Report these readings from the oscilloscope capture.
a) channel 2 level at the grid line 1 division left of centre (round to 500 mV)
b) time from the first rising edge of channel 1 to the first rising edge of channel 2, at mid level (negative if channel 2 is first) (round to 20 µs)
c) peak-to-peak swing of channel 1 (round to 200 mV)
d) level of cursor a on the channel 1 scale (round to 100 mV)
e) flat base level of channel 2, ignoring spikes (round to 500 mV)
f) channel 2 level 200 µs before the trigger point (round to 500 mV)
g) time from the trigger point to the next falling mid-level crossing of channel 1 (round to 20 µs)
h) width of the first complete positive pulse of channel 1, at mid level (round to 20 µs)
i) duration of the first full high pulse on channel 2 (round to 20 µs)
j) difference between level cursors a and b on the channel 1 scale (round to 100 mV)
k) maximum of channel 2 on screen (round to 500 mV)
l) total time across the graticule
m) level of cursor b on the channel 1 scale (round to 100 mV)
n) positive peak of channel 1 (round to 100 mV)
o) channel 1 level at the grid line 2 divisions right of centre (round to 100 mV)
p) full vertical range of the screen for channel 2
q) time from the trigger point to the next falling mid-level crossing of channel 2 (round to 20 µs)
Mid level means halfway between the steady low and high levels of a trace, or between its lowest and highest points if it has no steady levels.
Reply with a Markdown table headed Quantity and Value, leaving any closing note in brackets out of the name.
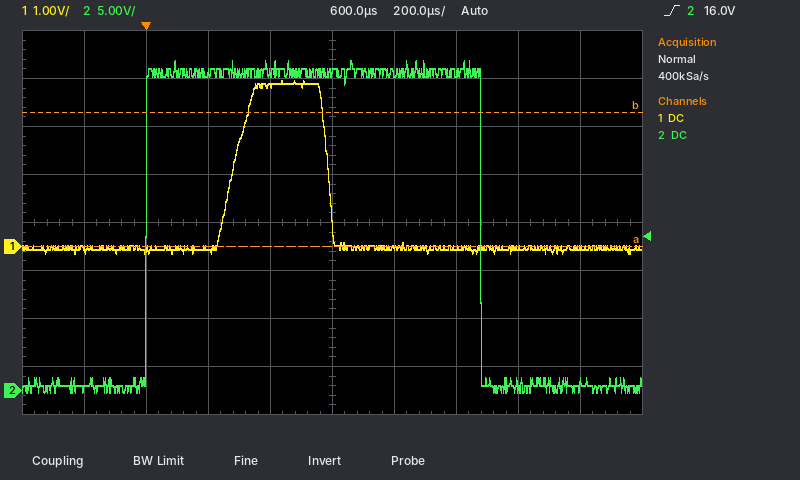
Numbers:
| Quantity | Value |
|---|---|
| channel 2 level at the grid line 1 division left of centre | 33.0 V |
| time from the first rising edge of channel 1 to the first rising edge of channel 2, at mid level (negative if channel 2 is first) | -280 µs |
| peak-to-peak swing of channel 1 | 3.6 V |
| level of cursor a on the channel 1 scale | 0.0 V |
| flat base level of channel 2, ignoring spikes | 500 mV |
| channel 2 level 200 µs before the trigger point | 0.0 V |
| time from the trigger point to the next falling mid-level crossing of channel 1 | 580 µs |
| width of the first complete positive pulse of channel 1, at mid level | 300 µs |
| duration of the first full high pulse on channel 2 | 1.08 ms |
| difference between level cursors a and b on the channel 1 scale | 2.8 V |
| maximum of channel 2 on screen | 34.5 V |
| total time across the graticule | 2 ms |
| level of cursor b on the channel 1 scale | 2.8 V |
| positive peak of channel 1 | 3.5 V |
| channel 1 level at the grid line 2 divisions right of centre | 0.0 V |
| full vertical range of the screen for channel 2 | 40 V |
| time from the trigger point to the next falling mid-level crossing of channel 2 | 1.08 ms |
